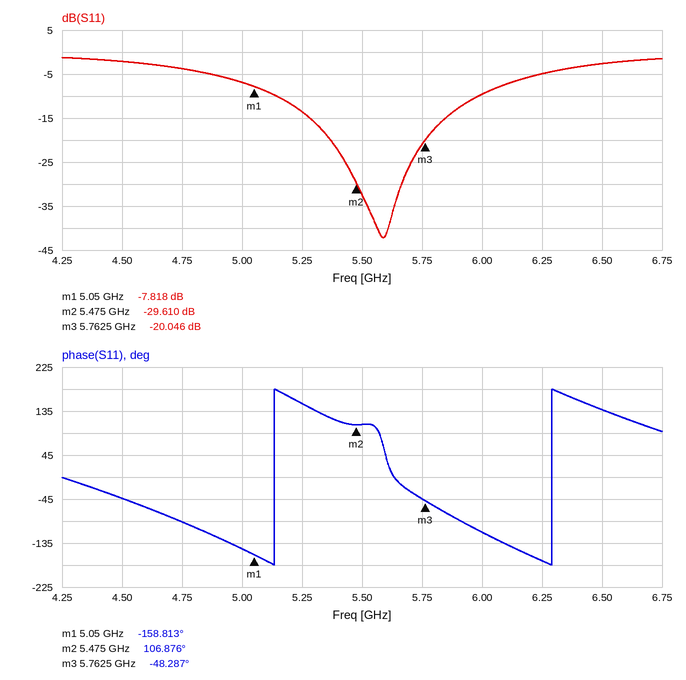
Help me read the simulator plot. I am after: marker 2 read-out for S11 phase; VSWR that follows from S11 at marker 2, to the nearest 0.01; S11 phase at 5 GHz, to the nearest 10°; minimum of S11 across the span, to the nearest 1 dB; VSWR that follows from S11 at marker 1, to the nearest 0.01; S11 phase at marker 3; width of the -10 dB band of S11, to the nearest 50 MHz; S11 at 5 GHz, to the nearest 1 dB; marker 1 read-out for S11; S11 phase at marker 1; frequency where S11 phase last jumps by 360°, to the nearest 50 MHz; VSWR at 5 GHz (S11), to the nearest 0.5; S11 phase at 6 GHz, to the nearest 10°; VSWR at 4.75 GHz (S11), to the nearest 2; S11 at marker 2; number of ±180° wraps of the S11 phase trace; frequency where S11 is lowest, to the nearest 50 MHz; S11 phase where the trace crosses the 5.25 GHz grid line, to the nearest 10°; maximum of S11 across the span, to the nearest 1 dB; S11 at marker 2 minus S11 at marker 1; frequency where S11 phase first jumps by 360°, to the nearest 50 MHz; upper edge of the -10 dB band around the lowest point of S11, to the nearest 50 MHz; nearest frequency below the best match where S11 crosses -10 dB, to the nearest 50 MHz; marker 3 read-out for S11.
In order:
106.876°
1.07
-150°
-42 dB
2.37
-48.287°
850 MHz
-7 dB
-7.818 dB
-158.813°
6.30 GHz
2.5
-110°
4
-29.610 dB
2
5.60 GHz
150°
-1 dB
-21.792 dB
5.15 GHz
6.00 GHz
5.15 GHz
-20.046 dB
